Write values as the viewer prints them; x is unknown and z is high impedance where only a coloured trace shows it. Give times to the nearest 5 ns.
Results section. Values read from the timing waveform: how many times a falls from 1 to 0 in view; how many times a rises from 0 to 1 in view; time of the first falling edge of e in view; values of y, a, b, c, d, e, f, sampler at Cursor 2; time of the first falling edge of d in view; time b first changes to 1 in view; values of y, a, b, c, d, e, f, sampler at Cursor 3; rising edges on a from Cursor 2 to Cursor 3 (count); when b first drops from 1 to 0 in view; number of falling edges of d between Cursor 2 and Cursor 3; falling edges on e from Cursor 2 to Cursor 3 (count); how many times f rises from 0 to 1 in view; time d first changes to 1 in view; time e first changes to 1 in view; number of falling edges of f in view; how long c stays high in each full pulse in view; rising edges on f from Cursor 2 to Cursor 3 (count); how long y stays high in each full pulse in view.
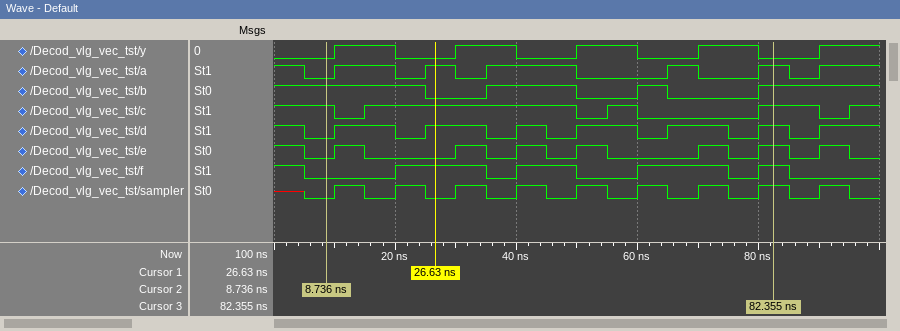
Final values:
6
6
5 ns
y=0, a=0, b=1, c=1, d=0, e=0, f=0, sampler=0
5 ns
35 ns
y=0, a=1, b=1, c=1, d=1, e=1, f=1, sampler=1
5
25 ns
5
5
4
10 ns
10 ns
5
35 ns, 5 ns, 10 ns
4
10 ns, 10 ns, 10 ns, 10 ns
